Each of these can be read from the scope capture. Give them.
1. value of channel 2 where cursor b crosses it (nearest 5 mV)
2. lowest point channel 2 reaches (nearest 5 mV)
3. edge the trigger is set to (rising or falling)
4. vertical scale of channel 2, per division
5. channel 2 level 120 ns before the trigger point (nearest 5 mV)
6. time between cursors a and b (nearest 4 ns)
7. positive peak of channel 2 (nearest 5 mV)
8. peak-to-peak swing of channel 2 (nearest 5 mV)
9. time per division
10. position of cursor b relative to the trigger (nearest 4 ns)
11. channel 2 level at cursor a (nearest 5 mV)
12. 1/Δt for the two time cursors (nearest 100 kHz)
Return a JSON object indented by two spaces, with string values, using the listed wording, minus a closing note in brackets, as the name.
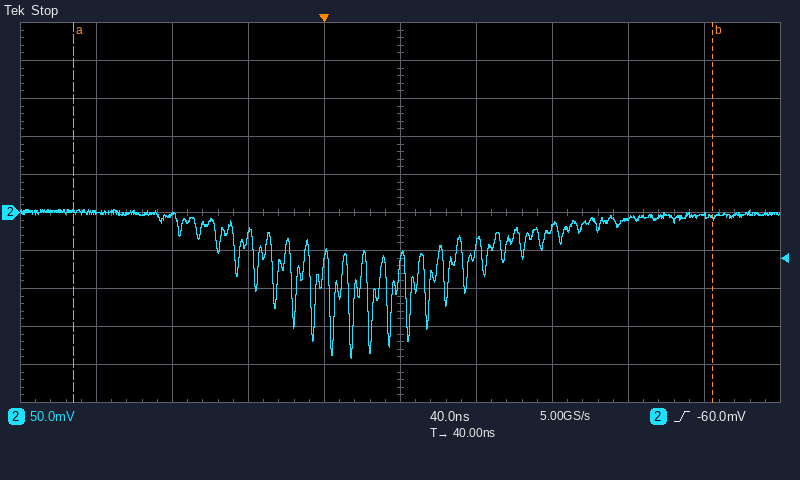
{
  "value of channel 2 where cursor b crosses it": "-5 mV",
  "lowest point channel 2 reaches": "-190 mV",
  "edge the trigger is set to": "rising",
  "vertical scale of channel 2, per division": "50 mV",
  "channel 2 level 120 ns before the trigger point": "0 mV",
  "time between cursors a and b": "336 ns",
  "positive peak of channel 2": "5 mV",
  "peak-to-peak swing of channel 2": "195 mV",
  "time per division": "40 ns",
  "position of cursor b relative to the trigger": "+204 ns",
  "channel 2 level at cursor a": "0 mV",
  "1/Δt for the two time cursors": "3.0 MHz"
}
